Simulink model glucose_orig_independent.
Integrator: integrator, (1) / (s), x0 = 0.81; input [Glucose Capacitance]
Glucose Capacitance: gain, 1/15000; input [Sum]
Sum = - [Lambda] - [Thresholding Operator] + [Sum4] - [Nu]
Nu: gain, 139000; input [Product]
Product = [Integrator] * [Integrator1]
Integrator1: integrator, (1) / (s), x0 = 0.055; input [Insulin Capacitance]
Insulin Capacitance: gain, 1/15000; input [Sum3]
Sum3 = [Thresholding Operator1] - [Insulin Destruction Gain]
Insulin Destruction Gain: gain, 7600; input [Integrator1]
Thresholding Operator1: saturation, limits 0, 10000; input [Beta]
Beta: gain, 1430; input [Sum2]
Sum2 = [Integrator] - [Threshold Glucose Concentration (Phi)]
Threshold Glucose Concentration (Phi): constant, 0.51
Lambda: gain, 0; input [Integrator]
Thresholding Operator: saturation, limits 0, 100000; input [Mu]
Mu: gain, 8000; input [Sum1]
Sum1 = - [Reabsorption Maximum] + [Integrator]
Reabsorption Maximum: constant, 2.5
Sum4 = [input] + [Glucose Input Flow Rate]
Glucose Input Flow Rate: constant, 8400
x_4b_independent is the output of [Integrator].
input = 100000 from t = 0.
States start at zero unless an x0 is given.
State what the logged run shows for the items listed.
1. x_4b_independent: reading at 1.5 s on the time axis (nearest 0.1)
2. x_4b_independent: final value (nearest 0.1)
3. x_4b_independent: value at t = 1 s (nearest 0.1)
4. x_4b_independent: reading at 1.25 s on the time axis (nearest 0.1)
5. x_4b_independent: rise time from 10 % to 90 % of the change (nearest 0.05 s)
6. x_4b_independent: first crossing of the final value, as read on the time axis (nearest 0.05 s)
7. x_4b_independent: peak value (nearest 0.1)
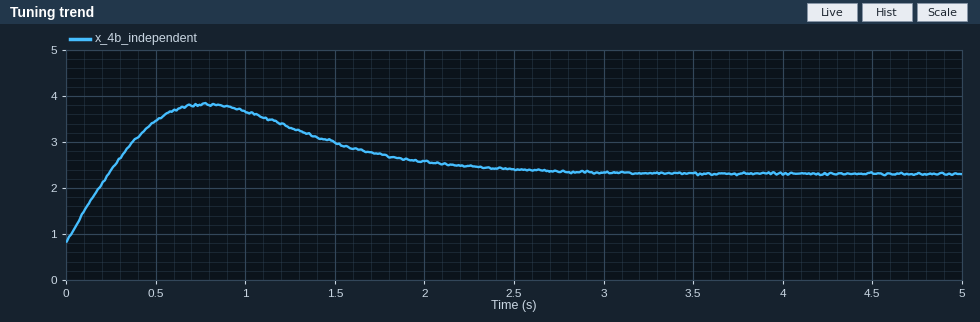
3.0
2.3
3.7
3.3
0.20 s
0.25 s
3.8
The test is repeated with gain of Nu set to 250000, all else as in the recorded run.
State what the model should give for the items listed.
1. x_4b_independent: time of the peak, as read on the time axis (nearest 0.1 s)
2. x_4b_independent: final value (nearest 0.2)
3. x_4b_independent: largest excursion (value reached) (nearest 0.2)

0.6 s
1.8
3.0
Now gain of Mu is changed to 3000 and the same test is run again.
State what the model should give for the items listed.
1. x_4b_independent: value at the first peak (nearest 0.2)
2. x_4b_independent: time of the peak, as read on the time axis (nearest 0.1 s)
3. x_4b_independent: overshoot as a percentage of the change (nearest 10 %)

4.0
0.8 s
110 %
